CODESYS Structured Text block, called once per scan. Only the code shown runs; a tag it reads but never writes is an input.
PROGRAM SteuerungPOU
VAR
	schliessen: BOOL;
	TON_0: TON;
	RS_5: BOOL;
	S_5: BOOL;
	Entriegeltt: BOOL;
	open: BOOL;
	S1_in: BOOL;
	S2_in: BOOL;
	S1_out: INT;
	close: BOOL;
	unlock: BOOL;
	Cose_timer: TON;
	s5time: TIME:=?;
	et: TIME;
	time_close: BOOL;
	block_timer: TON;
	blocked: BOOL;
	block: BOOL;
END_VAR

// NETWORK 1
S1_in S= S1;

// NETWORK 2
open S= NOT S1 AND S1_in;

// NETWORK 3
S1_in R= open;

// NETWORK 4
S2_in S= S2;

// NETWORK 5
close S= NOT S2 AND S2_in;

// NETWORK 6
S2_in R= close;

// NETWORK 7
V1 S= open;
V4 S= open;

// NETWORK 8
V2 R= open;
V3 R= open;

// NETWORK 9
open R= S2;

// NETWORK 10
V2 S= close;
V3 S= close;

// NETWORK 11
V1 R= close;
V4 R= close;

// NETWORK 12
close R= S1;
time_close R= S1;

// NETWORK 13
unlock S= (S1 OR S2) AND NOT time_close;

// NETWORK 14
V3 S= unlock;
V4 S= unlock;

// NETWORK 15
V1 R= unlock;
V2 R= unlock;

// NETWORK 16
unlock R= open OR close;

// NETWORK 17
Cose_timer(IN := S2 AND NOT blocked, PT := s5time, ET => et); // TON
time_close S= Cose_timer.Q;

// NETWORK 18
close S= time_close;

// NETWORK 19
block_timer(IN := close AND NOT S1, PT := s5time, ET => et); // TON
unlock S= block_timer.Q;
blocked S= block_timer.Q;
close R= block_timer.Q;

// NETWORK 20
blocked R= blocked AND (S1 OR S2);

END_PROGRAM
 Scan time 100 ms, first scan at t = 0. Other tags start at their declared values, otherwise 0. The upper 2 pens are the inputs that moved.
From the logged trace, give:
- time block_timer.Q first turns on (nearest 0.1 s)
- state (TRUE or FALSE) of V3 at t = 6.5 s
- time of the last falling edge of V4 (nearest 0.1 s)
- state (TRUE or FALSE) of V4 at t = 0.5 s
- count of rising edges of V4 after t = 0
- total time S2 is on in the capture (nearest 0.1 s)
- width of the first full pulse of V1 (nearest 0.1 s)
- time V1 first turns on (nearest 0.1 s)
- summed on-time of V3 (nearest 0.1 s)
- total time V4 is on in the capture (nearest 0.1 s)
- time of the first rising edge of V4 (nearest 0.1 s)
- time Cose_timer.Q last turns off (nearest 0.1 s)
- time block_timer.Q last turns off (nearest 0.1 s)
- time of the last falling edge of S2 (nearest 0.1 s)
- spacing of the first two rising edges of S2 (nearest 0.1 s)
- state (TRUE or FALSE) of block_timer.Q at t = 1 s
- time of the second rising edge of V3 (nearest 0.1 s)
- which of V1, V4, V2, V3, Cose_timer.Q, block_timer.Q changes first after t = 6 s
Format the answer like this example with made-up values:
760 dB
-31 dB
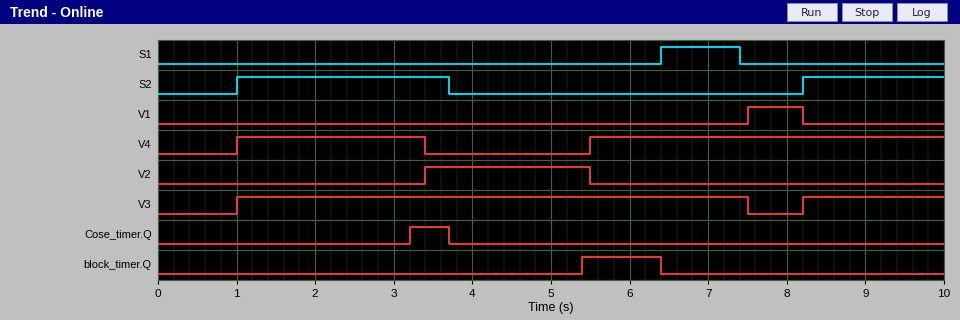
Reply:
5.4 s
TRUE
3.4 s
FALSE
2
4.5 s
0.7 s
7.5 s
8.3 s
6.9 s
1.0 s
3.7 s
6.4 s
3.7 s
7.2 s
FALSE
8.2 s
block_timer.Q
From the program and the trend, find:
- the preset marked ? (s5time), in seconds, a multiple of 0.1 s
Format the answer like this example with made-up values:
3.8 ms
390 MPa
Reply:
2.2 s
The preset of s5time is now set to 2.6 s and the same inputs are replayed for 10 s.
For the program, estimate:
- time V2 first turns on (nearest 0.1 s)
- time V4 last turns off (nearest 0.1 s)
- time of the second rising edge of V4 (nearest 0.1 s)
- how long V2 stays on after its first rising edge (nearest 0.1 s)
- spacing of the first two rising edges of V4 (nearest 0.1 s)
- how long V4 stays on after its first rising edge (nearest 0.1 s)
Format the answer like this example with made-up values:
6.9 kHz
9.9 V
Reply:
3.8 s
3.8 s
6.3 s
2.5 s
5.3 s
2.8 s
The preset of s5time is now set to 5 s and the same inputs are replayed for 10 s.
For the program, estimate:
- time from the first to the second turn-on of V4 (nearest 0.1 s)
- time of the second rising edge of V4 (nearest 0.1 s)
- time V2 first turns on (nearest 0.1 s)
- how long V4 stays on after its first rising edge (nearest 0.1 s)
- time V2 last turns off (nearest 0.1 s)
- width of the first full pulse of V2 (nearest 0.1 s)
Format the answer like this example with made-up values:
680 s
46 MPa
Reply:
5.4 s
6.4 s
3.8 s
2.8 s
6.4 s
2.6 s
